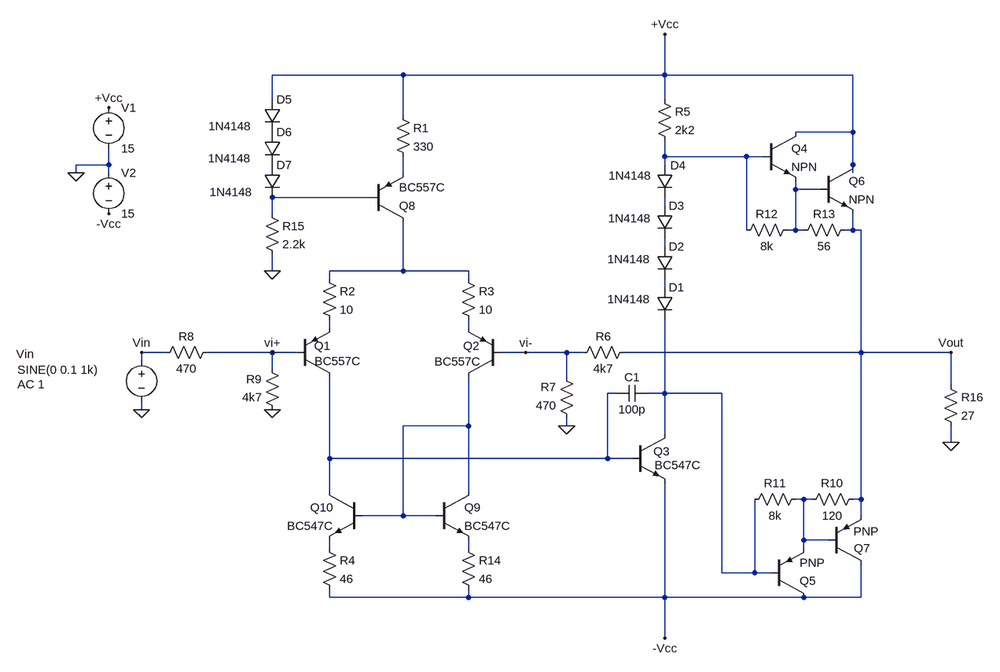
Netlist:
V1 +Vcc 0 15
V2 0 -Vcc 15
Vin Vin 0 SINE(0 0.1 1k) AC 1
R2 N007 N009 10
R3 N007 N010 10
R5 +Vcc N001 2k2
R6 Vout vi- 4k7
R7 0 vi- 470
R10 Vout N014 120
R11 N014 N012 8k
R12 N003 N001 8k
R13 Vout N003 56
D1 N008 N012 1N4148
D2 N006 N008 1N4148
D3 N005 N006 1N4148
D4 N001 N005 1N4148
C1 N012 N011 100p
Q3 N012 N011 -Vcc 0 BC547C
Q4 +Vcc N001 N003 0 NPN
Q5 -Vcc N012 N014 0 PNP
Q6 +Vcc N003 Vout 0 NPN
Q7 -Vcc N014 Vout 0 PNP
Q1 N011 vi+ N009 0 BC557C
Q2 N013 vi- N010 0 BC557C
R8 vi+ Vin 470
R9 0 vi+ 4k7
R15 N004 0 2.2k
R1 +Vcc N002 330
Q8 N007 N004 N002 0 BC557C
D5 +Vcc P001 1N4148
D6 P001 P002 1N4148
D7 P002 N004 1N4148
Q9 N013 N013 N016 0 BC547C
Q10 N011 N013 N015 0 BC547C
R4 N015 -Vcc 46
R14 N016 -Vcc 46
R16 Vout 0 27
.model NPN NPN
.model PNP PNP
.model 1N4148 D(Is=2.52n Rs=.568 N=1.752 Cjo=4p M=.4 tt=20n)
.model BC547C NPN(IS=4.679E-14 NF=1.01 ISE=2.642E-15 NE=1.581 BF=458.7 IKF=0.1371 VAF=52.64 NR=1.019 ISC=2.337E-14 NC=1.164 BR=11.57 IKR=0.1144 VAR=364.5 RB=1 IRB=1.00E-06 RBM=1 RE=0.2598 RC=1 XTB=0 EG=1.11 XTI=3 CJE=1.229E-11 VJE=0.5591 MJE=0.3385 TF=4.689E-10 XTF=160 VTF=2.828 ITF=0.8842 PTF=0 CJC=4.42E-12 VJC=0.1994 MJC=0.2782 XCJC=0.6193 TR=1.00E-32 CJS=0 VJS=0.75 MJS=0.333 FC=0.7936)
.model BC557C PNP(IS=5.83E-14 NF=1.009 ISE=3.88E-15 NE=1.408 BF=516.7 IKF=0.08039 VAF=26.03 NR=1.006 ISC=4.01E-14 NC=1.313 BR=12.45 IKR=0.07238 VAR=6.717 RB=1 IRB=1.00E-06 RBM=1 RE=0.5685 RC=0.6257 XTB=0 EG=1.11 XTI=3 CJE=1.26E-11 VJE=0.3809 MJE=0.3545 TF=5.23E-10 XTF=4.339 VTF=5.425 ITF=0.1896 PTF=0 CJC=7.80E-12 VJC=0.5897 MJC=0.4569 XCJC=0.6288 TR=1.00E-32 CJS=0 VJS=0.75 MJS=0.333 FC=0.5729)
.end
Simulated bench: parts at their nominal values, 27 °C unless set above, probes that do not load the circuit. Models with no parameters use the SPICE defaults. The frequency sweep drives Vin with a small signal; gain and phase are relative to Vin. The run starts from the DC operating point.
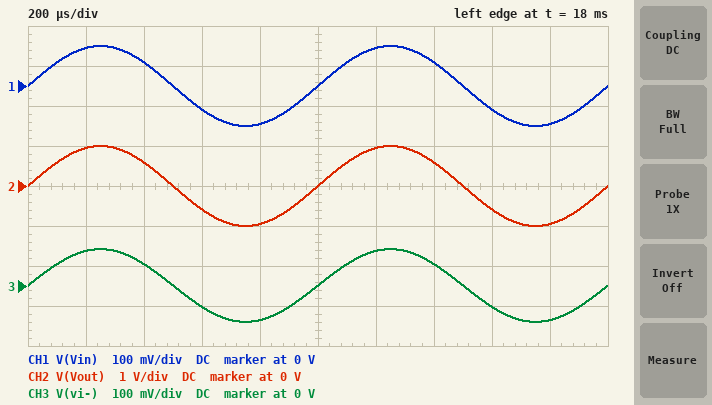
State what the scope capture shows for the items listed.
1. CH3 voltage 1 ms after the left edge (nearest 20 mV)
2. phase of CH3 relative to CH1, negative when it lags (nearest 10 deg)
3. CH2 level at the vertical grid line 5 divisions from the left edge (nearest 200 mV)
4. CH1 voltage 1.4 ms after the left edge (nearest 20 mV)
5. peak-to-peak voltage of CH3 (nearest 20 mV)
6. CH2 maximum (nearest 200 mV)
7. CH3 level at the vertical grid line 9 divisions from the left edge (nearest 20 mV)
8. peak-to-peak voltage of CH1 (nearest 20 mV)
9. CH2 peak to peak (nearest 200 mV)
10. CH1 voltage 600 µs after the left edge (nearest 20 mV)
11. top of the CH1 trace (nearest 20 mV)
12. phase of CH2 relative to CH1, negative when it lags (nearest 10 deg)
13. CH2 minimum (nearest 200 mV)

0 V
0 deg
0 V
60 mV
180 mV
1.0 V
-80 mV
200 mV
2.0 V
-60 mV
100 mV
0 deg
-1.0 V
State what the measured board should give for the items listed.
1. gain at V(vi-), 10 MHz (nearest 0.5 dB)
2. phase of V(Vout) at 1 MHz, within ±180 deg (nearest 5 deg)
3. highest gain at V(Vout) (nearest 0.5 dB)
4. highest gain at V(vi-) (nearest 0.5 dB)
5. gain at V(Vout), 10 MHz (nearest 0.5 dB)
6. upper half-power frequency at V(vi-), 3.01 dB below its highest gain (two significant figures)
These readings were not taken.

-13.0 dB
-25 deg
20.0 dB
-1.0 dB
5.0 dB
2.5 MHz
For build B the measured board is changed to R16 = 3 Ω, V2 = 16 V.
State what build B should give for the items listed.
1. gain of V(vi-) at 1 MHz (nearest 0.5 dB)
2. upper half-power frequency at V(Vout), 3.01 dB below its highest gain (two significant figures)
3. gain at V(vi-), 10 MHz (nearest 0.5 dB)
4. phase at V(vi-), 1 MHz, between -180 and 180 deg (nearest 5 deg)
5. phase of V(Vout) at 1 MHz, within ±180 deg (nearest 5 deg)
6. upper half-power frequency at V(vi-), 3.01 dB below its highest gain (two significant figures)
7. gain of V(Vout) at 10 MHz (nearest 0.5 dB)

-9.5 dB
470 kHz
-10.0 dB
-70 deg
-75 deg
440 kHz
-11.0 dB
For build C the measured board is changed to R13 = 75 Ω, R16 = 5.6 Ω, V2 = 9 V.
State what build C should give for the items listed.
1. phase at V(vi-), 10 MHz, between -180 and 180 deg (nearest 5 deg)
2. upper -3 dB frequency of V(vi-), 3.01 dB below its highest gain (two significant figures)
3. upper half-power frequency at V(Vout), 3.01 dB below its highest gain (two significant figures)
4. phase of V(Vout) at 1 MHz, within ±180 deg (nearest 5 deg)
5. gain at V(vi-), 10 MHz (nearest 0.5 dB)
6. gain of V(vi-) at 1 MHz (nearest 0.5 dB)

35 deg
600 kHz
650 kHz
-65 deg
-10.0 dB
-7.0 dB
